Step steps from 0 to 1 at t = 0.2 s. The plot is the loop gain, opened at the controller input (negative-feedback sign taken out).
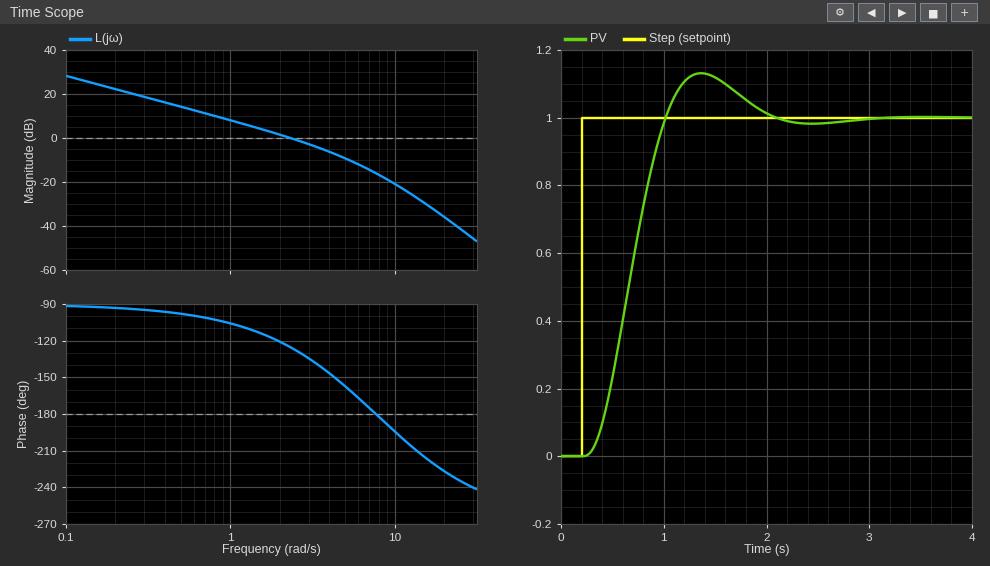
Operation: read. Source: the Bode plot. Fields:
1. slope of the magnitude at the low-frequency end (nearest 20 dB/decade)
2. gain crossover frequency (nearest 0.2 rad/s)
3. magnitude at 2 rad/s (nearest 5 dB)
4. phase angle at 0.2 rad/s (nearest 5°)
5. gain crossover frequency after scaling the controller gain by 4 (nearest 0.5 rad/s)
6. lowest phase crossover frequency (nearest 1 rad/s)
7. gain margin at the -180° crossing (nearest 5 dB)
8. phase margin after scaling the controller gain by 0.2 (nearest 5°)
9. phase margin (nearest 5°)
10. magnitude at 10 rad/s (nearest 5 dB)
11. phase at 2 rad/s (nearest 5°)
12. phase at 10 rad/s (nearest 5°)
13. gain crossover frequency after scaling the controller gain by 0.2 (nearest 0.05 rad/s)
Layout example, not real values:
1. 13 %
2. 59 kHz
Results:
1. -20 dB/decade
2. 2.4 rad/s
3. 0 dB
4. -95°
5. 6.0 rad/s
6. 8 rad/s
7. 15 dB
8. 80°
9. 55°
10. -20 dB
11. -120°
12. -195°
13. 0.50 rad/s
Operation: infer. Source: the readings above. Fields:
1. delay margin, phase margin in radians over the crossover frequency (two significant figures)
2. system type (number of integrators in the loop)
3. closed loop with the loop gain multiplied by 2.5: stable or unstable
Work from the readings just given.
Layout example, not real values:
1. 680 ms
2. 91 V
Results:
1. 0.40 s
2. 1
3. stable
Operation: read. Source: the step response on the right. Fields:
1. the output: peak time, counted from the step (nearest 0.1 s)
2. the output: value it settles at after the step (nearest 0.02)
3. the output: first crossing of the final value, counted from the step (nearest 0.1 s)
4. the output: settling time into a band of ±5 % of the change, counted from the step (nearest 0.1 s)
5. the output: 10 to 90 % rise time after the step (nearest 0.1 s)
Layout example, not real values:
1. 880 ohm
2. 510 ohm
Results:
1. 1.2 s
2. 1.00
3. 0.8 s
4. 1.6 s
5. 0.5 s
